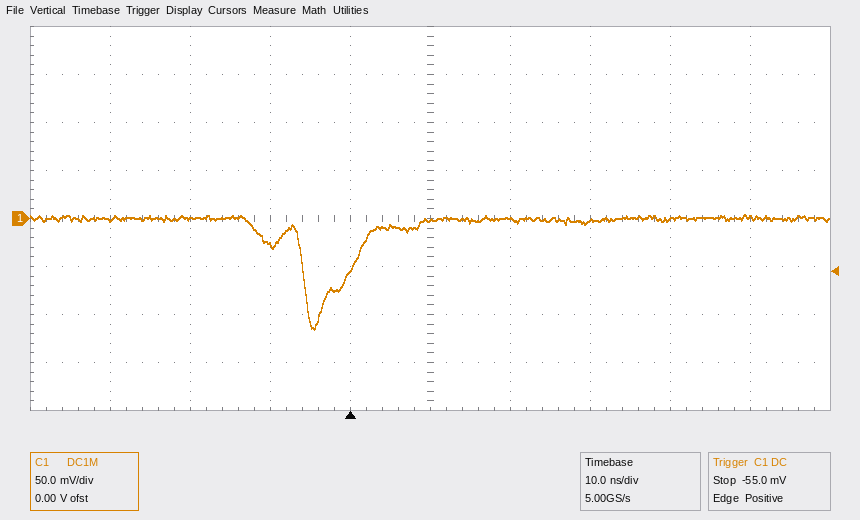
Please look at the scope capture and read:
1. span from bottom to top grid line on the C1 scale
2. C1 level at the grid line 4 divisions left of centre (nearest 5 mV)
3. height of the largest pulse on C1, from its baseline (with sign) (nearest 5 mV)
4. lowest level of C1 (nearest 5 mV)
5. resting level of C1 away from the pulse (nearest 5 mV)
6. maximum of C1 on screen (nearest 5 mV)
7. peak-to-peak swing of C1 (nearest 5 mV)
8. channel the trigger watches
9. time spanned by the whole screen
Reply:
400 mV
0 mV
-115 mV
-115 mV
0 mV
5 mV
120 mV
C1
100 ns
